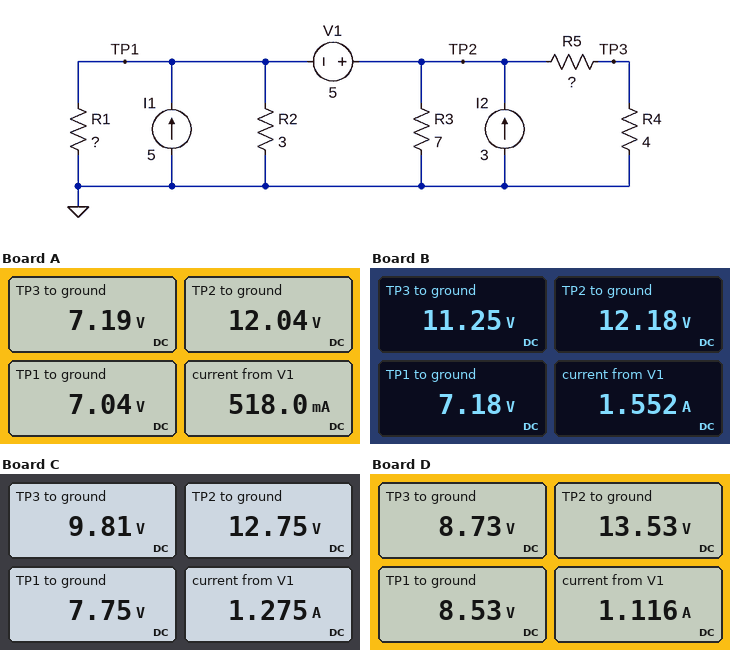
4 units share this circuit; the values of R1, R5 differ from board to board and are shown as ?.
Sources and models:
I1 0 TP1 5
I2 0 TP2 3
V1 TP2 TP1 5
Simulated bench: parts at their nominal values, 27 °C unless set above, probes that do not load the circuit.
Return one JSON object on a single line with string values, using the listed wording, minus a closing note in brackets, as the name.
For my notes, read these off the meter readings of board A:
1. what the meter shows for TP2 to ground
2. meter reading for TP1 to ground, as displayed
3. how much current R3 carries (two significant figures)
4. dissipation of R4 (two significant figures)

{"what the meter shows for TP2 to ground": "12.04 V", "meter reading for TP1 to ground, as displayed": "7.04 V", "how much current R3 carries": "1.7 A", "dissipation of R4": "13 W"}
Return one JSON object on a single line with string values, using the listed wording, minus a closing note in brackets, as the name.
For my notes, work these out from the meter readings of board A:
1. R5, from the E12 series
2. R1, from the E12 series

{"R5, from the E12 series": "2.7 Ω", "R1, from the E12 series": "3.3 Ω"}
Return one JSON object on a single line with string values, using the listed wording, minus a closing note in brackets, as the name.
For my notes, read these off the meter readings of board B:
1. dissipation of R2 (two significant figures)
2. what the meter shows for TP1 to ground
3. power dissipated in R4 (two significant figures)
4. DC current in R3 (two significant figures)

{"dissipation of R2": "17 W", "what the meter shows for TP1 to ground": "7.18 V", "power dissipated in R4": "32 W", "DC current in R3": "1.7 A"}
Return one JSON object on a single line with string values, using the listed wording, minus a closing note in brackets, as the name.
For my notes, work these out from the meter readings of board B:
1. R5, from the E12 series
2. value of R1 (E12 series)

{"R5, from the E12 series": "0.33 Ω", "value of R1": "6.8 Ω"}
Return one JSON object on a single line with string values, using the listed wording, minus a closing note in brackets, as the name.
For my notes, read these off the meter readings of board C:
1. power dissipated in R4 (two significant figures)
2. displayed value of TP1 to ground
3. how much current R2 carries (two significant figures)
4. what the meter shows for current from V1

{"power dissipated in R4": "24 W", "displayed value of TP1 to ground": "7.75 V", "how much current R2 carries": "2.6 A", "what the meter shows for current from V1": "1.275 A"}
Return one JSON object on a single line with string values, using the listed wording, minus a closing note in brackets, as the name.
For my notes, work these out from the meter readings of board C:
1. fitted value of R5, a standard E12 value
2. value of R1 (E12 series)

{"fitted value of R5, a standard E12 value": "1.2 Ω", "value of R1": "6.8 Ω"}
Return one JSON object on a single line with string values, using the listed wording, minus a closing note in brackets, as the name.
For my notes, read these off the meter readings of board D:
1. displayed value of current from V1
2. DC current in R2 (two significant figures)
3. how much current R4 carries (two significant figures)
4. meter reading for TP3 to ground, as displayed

{"displayed value of current from V1": "1.116 A", "DC current in R2": "2.8 A", "how much current R4 carries": "2.2 A", "meter reading for TP3 to ground, as displayed": "8.73 V"}
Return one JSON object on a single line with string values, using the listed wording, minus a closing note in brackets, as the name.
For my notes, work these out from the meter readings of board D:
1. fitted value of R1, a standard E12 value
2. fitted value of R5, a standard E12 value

{"fitted value of R1, a standard E12 value": "8.2 Ω", "fitted value of R5, a standard E12 value": "2.2 Ω"}
